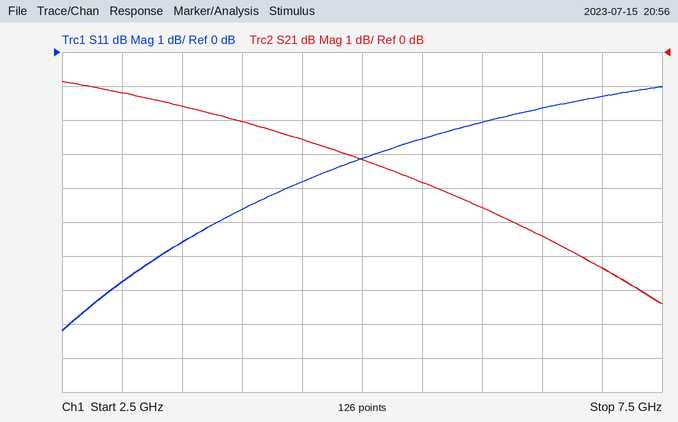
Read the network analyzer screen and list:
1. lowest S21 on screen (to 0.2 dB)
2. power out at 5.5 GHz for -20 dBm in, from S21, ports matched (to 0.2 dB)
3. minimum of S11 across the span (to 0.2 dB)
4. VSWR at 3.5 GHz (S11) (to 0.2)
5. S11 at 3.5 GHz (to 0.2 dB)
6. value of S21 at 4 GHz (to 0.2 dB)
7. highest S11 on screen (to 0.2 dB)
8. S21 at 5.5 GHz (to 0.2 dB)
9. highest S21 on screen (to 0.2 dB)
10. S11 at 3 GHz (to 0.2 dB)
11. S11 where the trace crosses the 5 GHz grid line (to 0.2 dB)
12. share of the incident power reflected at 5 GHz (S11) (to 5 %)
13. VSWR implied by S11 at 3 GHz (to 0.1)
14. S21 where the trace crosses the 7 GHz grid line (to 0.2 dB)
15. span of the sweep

-7.4 dB
-23.8 dBm
-8.2 dB
3.2
-5.6 dB
-2.0 dB
-1.0 dB
-3.8 dB
-0.8 dB
-6.8 dB
-3.2 dB
50 %
2.7
-6.4 dB
5 GHz
